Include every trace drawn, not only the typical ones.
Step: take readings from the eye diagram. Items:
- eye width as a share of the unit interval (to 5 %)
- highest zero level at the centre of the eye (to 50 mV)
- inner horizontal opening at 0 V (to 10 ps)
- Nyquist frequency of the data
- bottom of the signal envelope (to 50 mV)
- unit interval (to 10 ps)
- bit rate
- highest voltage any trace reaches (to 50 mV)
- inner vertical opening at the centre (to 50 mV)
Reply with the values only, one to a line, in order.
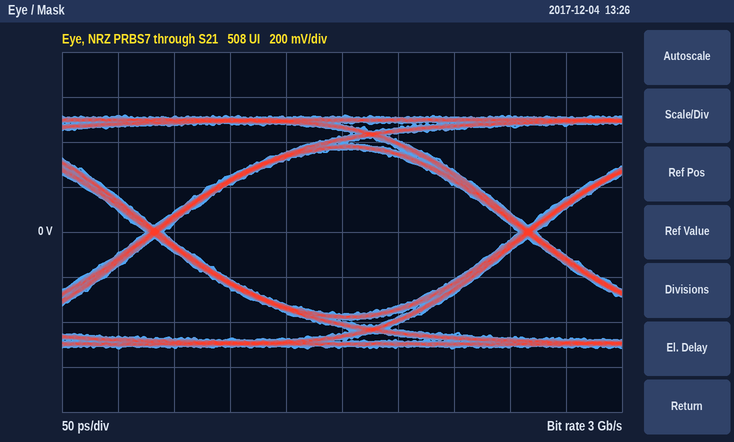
95 %
-350 mV
320 ps
1.5 GHz
-500 mV
330 ps
3 Gb/s
500 mV
750 mV
